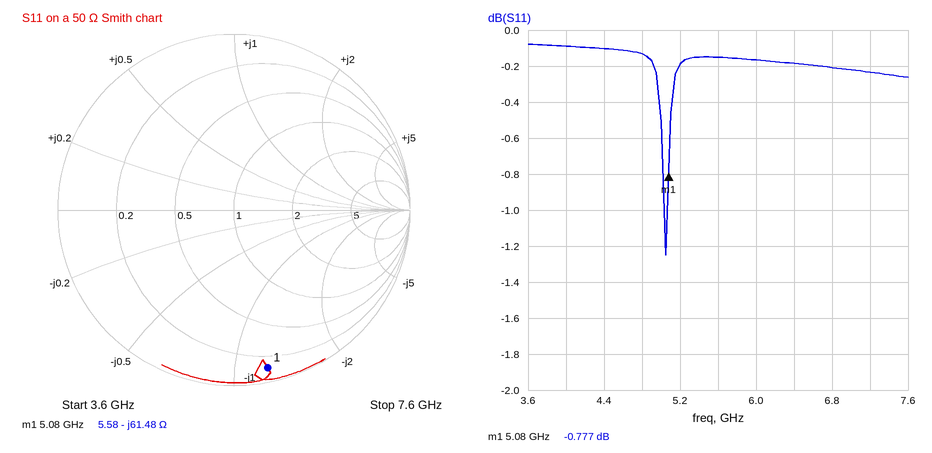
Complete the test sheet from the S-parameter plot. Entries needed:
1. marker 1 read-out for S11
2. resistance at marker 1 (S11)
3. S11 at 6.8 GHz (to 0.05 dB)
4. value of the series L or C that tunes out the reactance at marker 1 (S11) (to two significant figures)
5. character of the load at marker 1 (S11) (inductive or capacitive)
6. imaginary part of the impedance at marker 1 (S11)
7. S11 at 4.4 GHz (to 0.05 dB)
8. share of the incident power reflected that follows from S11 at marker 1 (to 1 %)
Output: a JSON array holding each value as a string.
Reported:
["-0.777 dB", "5.58 Ω", "-0.20 dB", "1.9 nH", "capacitive", "-61.48 Ω", "-0.10 dB", "84 %"]
